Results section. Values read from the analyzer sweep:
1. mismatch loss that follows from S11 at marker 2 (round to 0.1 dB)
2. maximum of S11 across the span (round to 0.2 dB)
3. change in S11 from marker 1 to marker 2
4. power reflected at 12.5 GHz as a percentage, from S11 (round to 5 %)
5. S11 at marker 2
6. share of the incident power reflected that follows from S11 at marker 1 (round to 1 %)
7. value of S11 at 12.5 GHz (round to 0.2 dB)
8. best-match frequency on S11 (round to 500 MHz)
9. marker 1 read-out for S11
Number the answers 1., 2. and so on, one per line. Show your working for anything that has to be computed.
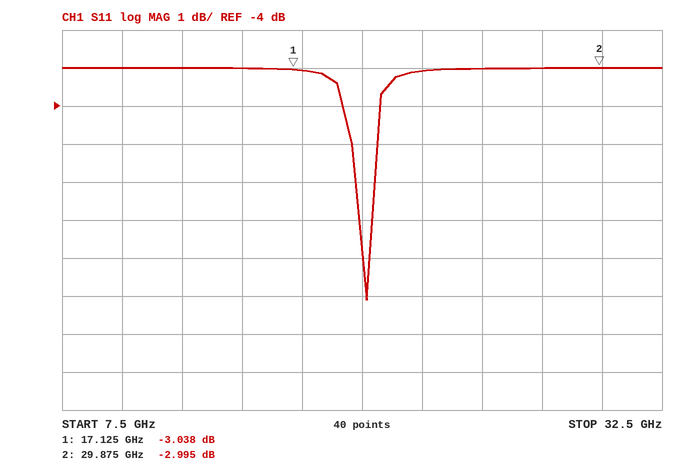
1. −10 log10(1 − 10^(-2.995/10)) ≈ 3.0 dB
2. -3.0 dB
3. -2.995 − (-3.038) = 0.043 dB
4. 10^(-3/10) ≈ 50 %
5. -2.995 dB
6. 10^(-3.038/10) ≈ 50 %
7. -3.0 dB
8. 20.0 GHz
9. -3.038 dB
